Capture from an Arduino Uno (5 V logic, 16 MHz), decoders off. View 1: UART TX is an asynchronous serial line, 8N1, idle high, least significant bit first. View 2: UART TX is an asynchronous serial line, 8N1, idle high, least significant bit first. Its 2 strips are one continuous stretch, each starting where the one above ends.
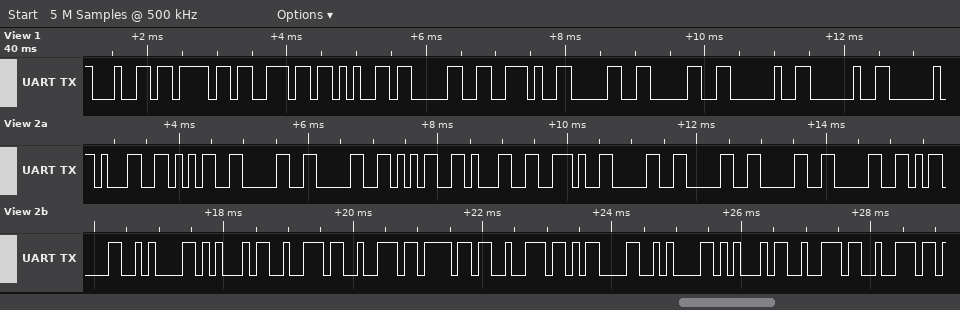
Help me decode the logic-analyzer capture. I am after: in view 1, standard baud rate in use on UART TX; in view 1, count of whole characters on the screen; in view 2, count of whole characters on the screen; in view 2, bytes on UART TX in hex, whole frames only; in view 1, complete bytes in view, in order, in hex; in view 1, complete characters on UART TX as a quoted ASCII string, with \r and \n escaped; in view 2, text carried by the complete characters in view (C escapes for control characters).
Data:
9600 baud
10
23
31 35 30 30 35 31 2E 30 30 30 30 0D 0A 45 72 72 6F 72 0D 0A 45 72 72
64 6F 6E 65 30 2E 30 30 20 20
"done0.00  "
"150051.0000\r\nError\r\nErr"
